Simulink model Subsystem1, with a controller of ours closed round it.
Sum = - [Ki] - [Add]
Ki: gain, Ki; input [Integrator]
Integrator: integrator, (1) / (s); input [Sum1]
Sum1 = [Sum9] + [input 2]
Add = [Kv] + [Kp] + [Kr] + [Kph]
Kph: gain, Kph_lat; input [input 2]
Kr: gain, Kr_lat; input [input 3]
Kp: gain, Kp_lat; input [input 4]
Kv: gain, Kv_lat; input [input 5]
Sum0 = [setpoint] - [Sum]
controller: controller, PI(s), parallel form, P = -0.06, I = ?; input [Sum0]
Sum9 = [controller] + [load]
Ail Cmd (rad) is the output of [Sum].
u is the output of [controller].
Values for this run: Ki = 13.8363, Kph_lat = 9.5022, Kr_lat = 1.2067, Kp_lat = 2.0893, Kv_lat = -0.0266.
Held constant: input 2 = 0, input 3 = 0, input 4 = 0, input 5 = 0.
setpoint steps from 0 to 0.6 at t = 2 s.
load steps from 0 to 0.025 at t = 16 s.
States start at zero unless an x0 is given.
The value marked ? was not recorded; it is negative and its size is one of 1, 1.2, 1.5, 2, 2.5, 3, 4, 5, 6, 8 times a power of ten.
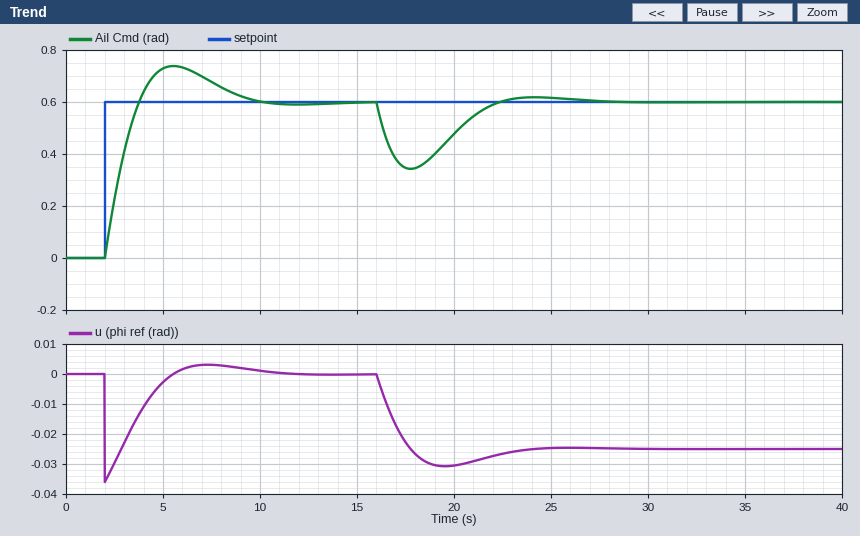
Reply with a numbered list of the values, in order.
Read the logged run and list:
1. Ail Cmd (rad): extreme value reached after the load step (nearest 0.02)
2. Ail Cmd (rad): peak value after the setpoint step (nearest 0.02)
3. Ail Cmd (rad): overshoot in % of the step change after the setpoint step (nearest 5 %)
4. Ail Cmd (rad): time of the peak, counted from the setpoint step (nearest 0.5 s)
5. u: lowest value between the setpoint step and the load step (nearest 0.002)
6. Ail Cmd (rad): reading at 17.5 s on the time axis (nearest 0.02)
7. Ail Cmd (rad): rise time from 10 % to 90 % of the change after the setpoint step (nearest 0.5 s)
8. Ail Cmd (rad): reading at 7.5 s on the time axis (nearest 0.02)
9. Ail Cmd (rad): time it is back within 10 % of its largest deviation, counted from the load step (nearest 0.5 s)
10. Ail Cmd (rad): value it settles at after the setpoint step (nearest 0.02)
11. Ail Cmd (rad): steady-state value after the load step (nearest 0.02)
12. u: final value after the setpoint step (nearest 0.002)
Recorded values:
1. 0.34
2. 0.74
3. 25 %
4. 3.5 s
5. -0.036
6. 0.34
7. 1.5 s
8. 0.68
9. 5.5 s
10. 0.60
11. 0.60
12. 0.000
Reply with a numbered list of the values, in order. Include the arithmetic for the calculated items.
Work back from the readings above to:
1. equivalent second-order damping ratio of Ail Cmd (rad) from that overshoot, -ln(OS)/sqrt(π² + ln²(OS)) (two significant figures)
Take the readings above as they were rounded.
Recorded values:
1. ln(0.25) = -1.386; 1.386 / sqrt(9.870 + 1.922) = 0.40
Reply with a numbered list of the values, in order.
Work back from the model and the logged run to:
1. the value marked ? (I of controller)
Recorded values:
1. -0.03
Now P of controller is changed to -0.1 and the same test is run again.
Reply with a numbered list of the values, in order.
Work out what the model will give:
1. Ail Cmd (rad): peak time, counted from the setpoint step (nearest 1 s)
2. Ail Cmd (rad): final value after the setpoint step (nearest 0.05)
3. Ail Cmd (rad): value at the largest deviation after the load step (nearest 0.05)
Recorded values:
1. 3 s
2. 0.60
3. 0.40
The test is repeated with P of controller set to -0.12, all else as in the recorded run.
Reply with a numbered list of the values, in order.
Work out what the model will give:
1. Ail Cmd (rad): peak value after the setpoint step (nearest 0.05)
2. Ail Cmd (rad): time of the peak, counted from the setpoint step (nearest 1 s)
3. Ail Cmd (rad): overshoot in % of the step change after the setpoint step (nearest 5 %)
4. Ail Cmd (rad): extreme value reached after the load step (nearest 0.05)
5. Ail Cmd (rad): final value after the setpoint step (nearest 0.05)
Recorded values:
1. 0.65
2. 3 s
3. 10 %
4. 0.45
5. 0.60
